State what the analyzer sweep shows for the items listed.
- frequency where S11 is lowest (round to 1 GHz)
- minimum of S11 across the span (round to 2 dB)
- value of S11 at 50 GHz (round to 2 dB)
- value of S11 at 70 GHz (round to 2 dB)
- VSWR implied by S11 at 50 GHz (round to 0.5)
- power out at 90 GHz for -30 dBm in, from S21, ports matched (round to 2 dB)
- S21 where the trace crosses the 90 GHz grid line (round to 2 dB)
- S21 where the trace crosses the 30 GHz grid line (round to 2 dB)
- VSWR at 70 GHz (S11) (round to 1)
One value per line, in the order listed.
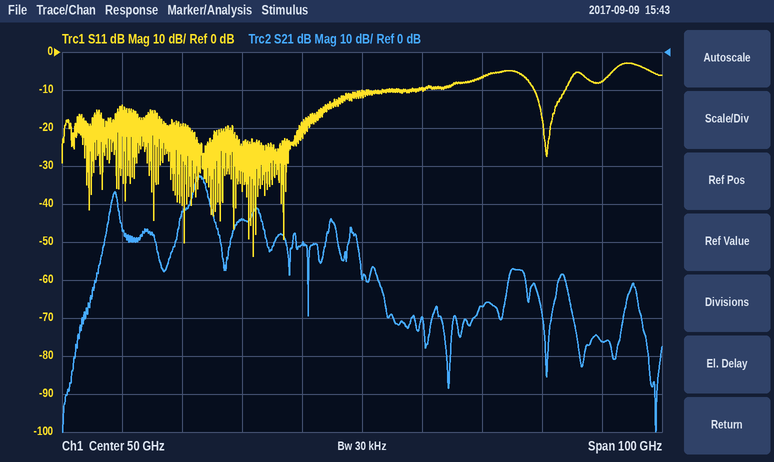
32 GHz
-54 dB
-10 dB
-6 dB
2.0
-106 dBm
-76 dB
-44 dB
3
